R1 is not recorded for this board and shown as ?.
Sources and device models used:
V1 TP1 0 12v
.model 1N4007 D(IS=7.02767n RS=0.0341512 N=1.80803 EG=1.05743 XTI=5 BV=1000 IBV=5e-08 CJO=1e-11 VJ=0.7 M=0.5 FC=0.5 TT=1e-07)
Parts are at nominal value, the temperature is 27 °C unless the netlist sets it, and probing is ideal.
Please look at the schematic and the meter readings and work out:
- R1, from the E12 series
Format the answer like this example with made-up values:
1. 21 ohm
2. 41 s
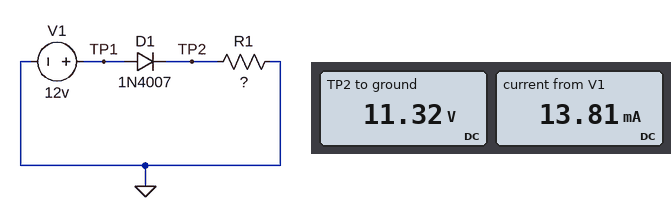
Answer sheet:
1. 820 Ω
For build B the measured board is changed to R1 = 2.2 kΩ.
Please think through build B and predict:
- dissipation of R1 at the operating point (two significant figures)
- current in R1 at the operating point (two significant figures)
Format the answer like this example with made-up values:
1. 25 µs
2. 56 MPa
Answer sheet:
1. 59 mW
2. 5.2 mA
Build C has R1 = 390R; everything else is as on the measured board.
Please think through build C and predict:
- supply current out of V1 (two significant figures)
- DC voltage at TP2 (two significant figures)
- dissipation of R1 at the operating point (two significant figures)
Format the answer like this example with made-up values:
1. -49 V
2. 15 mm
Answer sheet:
1. 29 mA
2. 11 V
3. 330 mW
